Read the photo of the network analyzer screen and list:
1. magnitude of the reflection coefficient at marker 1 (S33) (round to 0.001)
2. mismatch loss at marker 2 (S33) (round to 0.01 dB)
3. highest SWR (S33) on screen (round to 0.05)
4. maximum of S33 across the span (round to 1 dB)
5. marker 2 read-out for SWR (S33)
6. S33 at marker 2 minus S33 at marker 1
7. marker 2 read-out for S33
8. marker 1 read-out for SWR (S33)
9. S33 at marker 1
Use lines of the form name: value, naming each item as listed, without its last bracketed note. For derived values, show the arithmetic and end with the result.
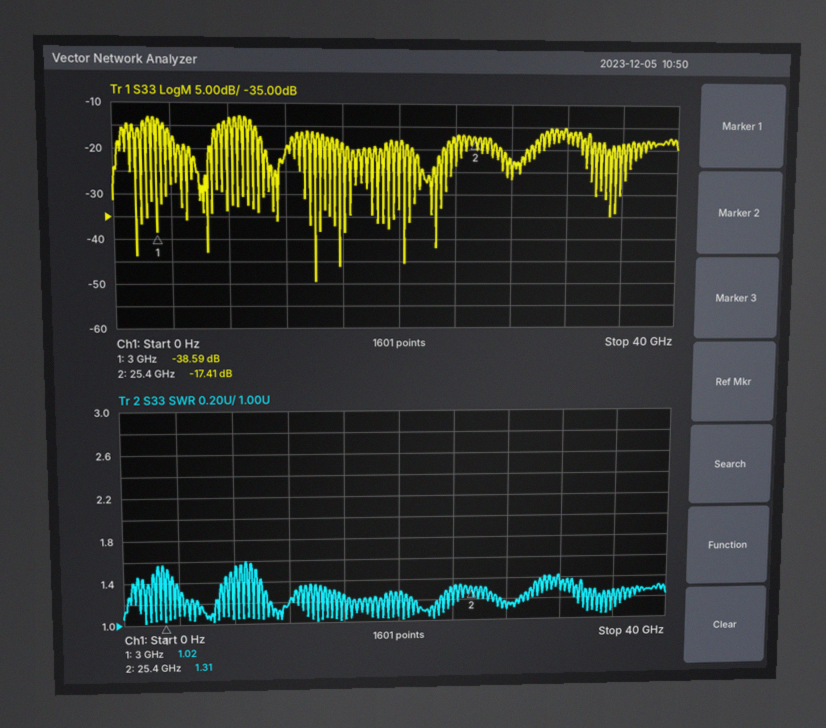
magnitude of the reflection coefficient at marker 1 (S33): 10^(-38.59/20) ≈ 0.012
mismatch loss at marker 2 (S33): −10 log10(1 − 10^(-17.41/10)) ≈ 0.08 dB
highest SWR (S33) on screen: 1.60
maximum of S33 across the span: -13 dB
marker 2 read-out for SWR: 1.31
S33 at marker 2 minus S33 at marker 1: -17.41 − (-38.59) = 21.18 dB
marker 2 read-out for S33: -17.41 dB
marker 1 read-out for SWR: 1.02
S33 at marker 1: -38.59 dB
